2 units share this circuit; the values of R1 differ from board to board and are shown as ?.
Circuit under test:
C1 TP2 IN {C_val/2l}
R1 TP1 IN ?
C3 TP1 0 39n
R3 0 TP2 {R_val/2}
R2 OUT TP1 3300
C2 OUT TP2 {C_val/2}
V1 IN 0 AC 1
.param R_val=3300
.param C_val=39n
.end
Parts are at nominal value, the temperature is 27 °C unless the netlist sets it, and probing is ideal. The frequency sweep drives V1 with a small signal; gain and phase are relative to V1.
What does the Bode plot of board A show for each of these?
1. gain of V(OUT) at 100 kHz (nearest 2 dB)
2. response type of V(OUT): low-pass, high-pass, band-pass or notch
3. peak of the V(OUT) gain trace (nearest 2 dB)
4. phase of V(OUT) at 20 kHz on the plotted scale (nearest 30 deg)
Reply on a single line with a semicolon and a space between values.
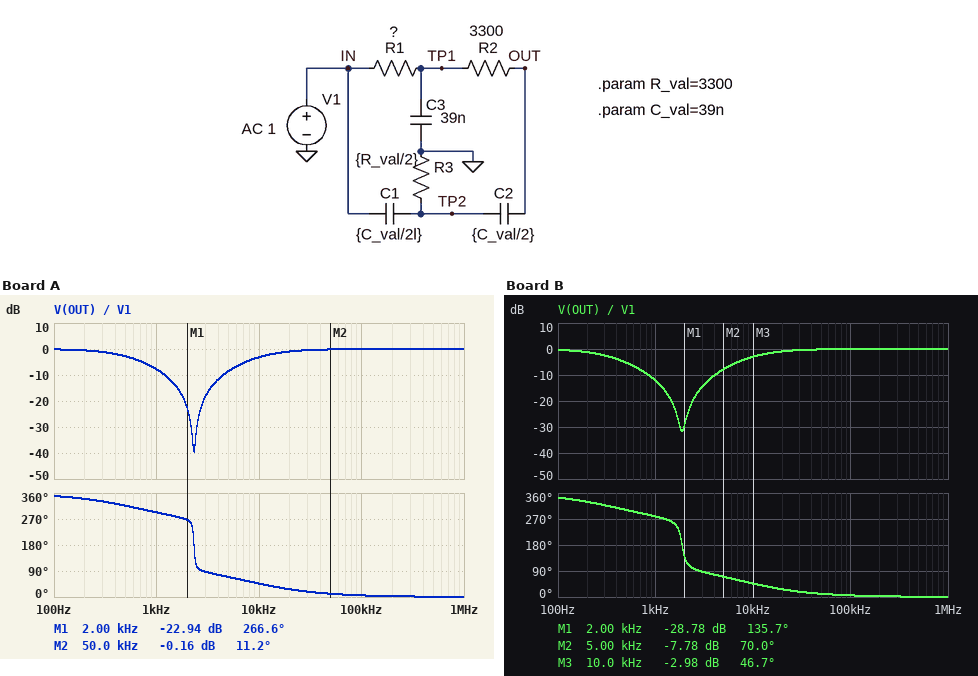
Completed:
0 dB; notch; 0 dB; 30 deg
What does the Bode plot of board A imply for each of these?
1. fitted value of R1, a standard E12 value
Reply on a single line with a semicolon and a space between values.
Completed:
3.9 kΩ
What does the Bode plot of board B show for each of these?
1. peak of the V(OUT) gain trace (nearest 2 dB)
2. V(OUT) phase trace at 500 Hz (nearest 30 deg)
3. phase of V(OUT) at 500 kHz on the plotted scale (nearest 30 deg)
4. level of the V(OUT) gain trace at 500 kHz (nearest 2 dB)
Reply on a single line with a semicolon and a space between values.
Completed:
0 dB; 300 deg; 0 deg; 0 dB
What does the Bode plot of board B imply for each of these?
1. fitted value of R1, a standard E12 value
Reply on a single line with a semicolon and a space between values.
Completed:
6.8 kΩ
